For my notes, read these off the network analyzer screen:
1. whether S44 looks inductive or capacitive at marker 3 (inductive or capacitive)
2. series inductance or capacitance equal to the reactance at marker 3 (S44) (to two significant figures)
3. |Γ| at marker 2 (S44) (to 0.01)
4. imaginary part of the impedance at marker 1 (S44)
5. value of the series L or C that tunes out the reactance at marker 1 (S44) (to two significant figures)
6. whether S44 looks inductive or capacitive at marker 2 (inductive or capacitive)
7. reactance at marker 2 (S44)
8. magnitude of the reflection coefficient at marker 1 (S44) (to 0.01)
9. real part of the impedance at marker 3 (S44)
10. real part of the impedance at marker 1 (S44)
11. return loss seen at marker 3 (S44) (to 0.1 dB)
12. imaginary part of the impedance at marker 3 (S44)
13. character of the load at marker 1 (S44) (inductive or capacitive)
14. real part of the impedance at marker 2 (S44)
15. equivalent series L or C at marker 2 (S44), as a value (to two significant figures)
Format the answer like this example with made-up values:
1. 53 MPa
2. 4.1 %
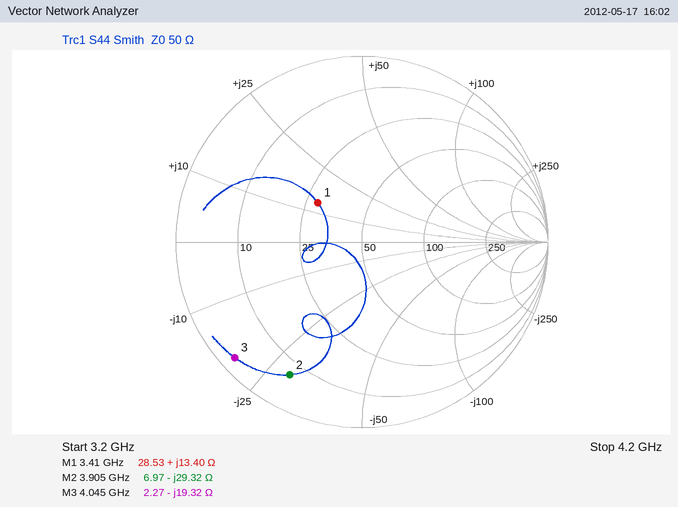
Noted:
1. capacitive
2. 2.0 pF
3. 0.81
4. +13.40 Ω
5. 3.5 pF
6. capacitive
7. -29.32 Ω
8. 0.32
9. 2.27 Ω
10. 28.53 Ω
11. 0.7 dB
12. -19.32 Ω
13. inductive
14. 6.97 Ω
15. 1.4 pF
